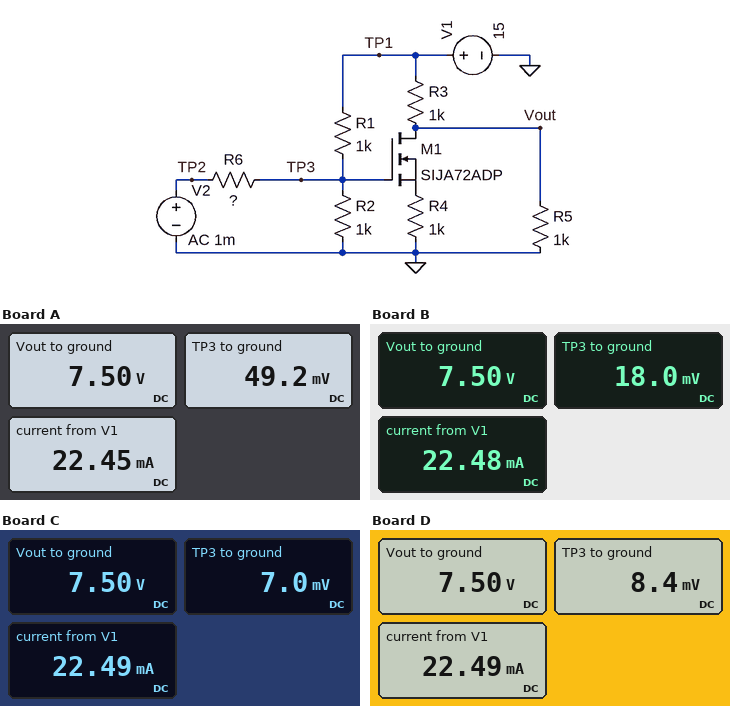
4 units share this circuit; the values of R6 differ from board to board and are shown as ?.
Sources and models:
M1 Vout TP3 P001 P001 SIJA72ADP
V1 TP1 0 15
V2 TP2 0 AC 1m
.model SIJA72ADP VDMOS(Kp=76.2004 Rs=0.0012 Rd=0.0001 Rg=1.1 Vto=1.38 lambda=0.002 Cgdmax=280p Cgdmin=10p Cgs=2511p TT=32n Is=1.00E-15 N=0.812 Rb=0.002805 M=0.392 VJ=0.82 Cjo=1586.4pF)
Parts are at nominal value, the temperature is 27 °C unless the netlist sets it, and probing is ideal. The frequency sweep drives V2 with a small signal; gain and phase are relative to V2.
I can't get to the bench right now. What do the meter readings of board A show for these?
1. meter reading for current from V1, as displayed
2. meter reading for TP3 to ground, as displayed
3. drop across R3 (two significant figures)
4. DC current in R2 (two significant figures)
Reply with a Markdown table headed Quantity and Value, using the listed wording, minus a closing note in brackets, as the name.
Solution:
| Quantity | Value |
|---|---|
| meter reading for current from V1, as displayed | 22.45 mA |
| meter reading for TP3 to ground, as displayed | 49.2 mV |
| drop across R3 | 7.5 V |
| DC current in R2 | 49 µA |
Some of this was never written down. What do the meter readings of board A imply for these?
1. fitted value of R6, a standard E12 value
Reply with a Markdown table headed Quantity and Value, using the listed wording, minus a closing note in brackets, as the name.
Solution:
| Quantity | Value |
|---|---|
| fitted value of R6, a standard E12 value | 3.3 Ω |
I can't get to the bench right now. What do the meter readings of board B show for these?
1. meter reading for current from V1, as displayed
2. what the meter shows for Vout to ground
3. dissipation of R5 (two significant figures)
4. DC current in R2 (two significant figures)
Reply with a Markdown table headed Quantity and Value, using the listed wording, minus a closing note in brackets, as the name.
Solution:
| Quantity | Value |
|---|---|
| meter reading for current from V1, as displayed | 22.48 mA |
| what the meter shows for Vout to ground | 7.50 V |
| dissipation of R5 | 56 mW |
| DC current in R2 | 18 µA |
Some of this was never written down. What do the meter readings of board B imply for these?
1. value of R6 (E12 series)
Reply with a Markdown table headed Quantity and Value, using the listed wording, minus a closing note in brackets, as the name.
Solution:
| Quantity | Value |
|---|---|
| value of R6 | 1.2 Ω |
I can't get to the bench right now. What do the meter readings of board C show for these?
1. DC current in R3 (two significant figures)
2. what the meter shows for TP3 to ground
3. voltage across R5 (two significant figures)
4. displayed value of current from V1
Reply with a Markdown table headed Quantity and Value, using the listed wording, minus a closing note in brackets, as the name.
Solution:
| Quantity | Value |
|---|---|
| DC current in R3 | 7.5 mA |
| what the meter shows for TP3 to ground | 7.0 mV |
| voltage across R5 | 7.5 V |
| displayed value of current from V1 | 22.49 mA |
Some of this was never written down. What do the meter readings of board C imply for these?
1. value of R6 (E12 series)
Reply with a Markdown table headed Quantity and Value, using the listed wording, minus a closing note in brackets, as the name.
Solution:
| Quantity | Value |
|---|---|
| value of R6 | 0.47 Ω |
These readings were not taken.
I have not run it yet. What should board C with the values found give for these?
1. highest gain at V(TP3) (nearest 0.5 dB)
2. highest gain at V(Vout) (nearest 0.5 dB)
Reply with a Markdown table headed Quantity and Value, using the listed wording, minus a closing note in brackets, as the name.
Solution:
| Quantity | Value |
|---|---|
| highest gain at V(TP3) | 0 dB |
| highest gain at V(Vout) | 0 dB |
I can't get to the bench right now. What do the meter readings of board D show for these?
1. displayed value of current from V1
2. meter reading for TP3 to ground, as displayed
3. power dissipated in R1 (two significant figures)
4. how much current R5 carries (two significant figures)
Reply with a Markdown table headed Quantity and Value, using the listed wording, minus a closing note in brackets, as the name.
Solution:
| Quantity | Value |
|---|---|
| displayed value of current from V1 | 22.49 mA |
| meter reading for TP3 to ground, as displayed | 8.4 mV |
| power dissipated in R1 | 220 mW |
| how much current R5 carries | 7.5 mA |
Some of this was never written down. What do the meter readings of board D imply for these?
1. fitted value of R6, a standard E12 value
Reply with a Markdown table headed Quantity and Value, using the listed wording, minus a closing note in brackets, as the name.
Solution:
| Quantity | Value |
|---|---|
| fitted value of R6, a standard E12 value | 0.56 Ω |
